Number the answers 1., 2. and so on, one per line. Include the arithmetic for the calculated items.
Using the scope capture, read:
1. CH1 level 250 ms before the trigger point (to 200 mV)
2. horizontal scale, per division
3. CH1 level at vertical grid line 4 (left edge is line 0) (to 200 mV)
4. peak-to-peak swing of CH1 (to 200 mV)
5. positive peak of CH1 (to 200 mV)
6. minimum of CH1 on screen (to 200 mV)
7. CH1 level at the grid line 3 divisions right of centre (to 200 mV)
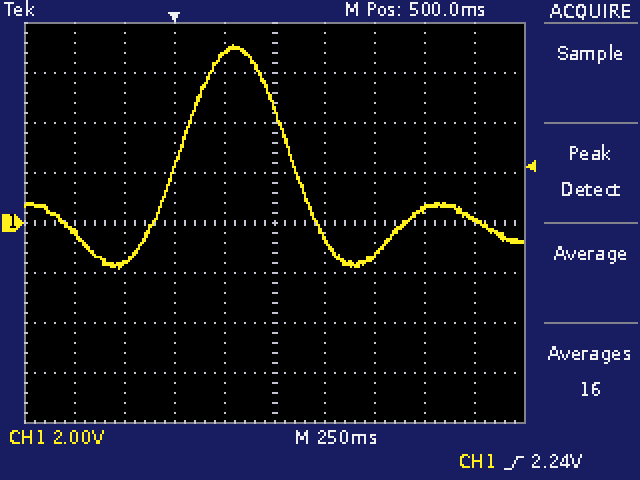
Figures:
1. -1.6 V
2. 250 ms
3. 6.8 V
4. 7.2 V − (-1.8 V) = 9.0 V
5. 7.2 V
6. -1.8 V
7. 600 mV
